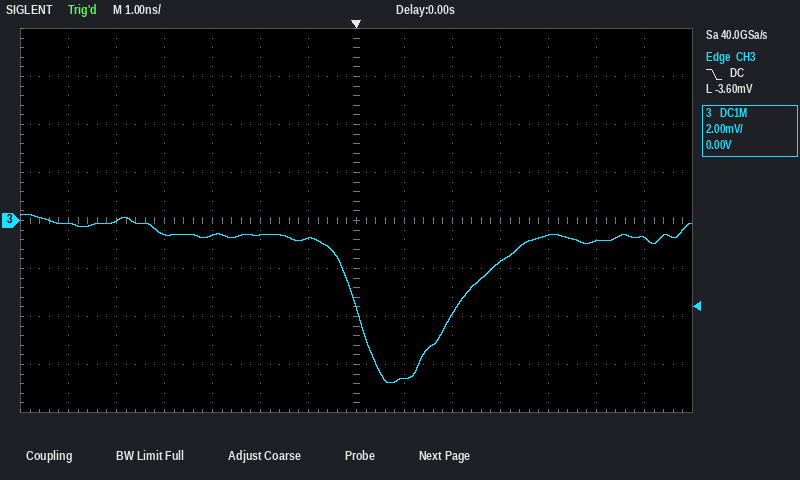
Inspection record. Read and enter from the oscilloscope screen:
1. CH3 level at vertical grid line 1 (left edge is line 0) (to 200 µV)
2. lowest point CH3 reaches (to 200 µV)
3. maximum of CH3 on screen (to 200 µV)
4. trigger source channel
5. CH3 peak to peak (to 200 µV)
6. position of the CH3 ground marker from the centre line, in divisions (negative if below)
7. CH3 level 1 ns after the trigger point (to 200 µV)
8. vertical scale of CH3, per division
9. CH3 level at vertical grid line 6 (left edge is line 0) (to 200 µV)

-200 µV
-6.8 mV
200 µV
CH3
7.0 mV
0.0 div
-6.6 mV
2 mV
-800 µV
